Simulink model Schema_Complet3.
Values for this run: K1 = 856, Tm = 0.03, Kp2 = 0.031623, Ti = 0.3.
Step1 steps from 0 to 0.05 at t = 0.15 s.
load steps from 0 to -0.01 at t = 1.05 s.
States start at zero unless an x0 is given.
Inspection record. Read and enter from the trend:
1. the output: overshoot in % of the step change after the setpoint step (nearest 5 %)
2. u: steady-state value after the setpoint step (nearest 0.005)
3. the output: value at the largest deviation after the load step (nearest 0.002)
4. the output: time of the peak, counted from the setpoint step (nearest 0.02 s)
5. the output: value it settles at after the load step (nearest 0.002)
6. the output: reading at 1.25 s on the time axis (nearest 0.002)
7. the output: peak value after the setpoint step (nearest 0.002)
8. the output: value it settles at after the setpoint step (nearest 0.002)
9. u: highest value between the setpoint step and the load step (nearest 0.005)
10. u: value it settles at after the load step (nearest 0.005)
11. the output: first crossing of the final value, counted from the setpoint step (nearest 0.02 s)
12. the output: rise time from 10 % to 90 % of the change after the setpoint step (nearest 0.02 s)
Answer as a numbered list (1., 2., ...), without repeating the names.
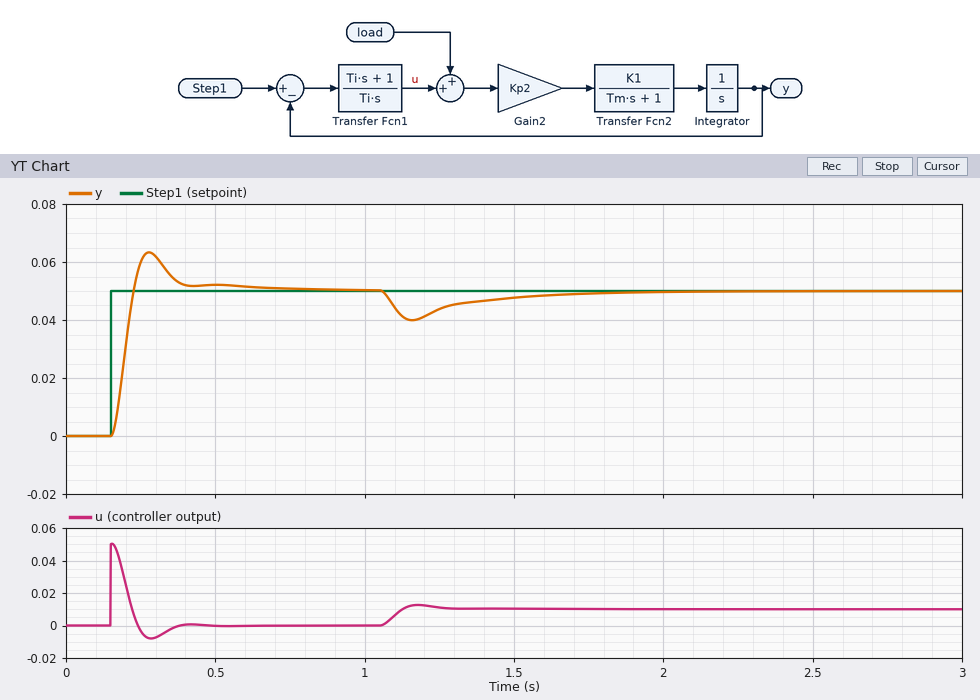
1. 25 %
2. 0.000
3. 0.040
4. 0.12 s
5. 0.050
6. 0.044
7. 0.064
8. 0.050
9. 0.050
10. 0.010
11. 0.08 s
12. 0.06 s
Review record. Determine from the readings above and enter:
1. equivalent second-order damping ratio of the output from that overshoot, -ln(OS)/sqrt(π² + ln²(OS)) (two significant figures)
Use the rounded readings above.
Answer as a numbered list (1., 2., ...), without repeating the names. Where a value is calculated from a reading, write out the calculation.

1. ln(0.25) = -1.386; 1.386 / sqrt(9.870 + 1.922) = 0.40
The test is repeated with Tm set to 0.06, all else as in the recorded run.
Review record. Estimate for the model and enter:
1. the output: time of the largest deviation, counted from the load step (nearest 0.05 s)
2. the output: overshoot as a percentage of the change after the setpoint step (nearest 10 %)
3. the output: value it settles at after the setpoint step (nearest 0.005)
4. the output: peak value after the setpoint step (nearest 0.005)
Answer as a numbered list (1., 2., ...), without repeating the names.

1. 0.15 s
2. 50 %
3. 0.050
4. 0.075
